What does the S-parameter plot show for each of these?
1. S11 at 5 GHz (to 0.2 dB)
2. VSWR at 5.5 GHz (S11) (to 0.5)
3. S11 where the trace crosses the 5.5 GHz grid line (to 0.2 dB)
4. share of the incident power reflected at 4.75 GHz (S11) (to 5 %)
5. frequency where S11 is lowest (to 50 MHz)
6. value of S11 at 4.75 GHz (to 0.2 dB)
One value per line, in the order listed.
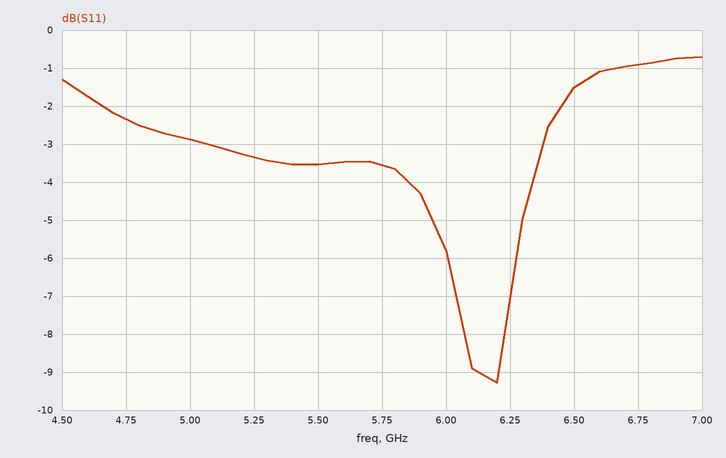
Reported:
-2.8 dB
5.0
-3.6 dB
60 %
6.20 GHz
-2.4 dB
